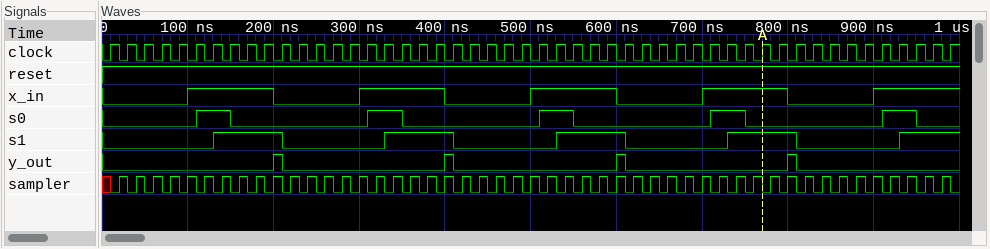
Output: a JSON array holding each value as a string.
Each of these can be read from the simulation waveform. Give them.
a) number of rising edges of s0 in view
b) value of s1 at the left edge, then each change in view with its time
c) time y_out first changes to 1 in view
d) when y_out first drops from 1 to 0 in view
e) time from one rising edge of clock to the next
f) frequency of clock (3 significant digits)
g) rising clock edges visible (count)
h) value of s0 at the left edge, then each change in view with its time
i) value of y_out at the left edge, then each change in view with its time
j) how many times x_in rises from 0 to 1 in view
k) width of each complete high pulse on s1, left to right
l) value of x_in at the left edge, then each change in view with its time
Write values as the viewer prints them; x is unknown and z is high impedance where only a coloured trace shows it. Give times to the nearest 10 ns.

["5", "0, 1 at 130 ns, 0 at 210 ns, 1 at 330 ns, 0 at 410 ns, 1 at 530 ns, 0 at 610 ns, 1 at 730 ns, 0 at 810 ns, 1 at 930 ns", "200 ns", "210 ns", "20 ns", "50.0 MHz", "50", "0, 1 at 110 ns, 0 at 150 ns, 1 at 310 ns, 0 at 350 ns, 1 at 510 ns, 0 at 550 ns, 1 at 710 ns, 0 at 750 ns, 1 at 910 ns, 0 at 950 ns", "0, 1 at 200 ns, 0 at 210 ns, 1 at 400 ns, 0 at 410 ns, 1 at 600 ns, 0 at 610 ns, 1 at 800 ns, 0 at 810 ns", "5", "80 ns, 80 ns, 80 ns, 80 ns", "0, 1 at 100 ns, 0 at 200 ns, 1 at 300 ns, 0 at 400 ns, 1 at 500 ns, 0 at 600 ns, 1 at 700 ns, 0 at 800 ns, 1 at 900 ns"]
